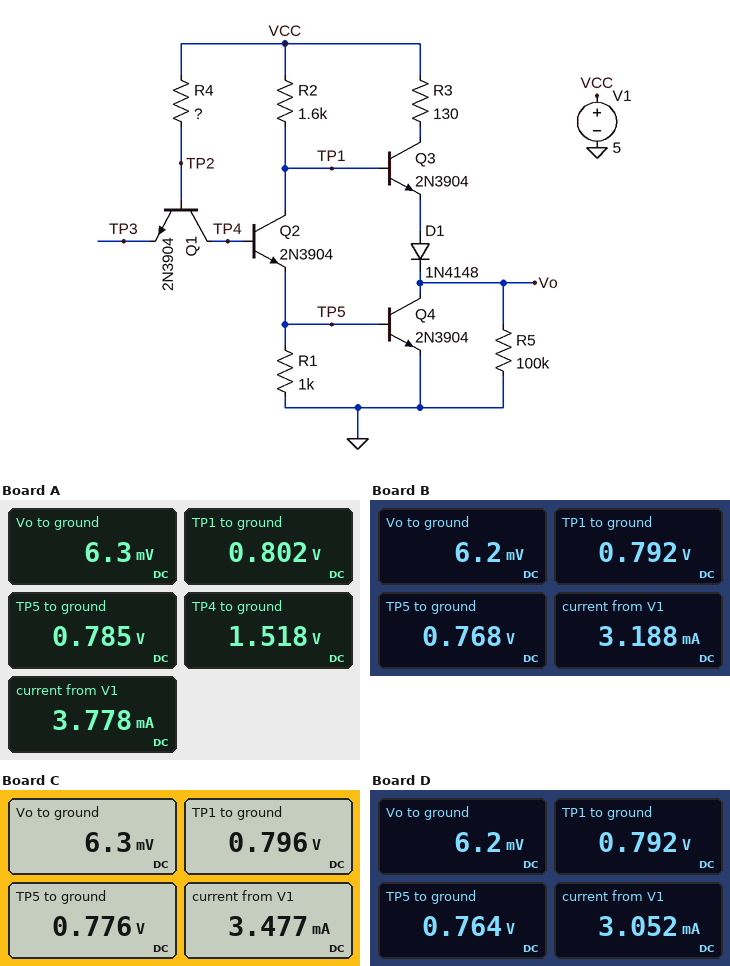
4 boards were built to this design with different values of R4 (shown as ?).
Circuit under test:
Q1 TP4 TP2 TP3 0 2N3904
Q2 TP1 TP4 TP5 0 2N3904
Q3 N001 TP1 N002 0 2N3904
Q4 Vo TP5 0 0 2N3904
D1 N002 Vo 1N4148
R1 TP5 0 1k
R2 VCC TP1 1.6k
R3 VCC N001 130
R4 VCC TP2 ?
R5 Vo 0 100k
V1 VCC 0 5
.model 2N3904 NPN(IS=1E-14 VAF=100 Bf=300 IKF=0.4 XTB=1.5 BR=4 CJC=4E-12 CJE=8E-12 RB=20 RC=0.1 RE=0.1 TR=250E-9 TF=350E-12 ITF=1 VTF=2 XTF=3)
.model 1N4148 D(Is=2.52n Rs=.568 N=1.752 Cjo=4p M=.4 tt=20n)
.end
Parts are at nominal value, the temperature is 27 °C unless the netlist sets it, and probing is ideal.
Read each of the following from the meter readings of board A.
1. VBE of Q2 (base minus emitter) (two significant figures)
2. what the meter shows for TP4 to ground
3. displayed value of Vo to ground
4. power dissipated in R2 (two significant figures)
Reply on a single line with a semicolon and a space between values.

730 mV; 1.518 V; 6.3 mV; 11 mW
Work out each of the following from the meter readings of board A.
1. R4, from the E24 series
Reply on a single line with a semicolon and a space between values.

2.4 kΩ
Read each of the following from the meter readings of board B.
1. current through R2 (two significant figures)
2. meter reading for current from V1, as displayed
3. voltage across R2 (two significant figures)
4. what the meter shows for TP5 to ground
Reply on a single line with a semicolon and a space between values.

2.6 mA; 3.188 mA; 4.2 V; 0.768 V
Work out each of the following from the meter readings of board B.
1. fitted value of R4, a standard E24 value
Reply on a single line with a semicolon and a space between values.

5.1 kΩ
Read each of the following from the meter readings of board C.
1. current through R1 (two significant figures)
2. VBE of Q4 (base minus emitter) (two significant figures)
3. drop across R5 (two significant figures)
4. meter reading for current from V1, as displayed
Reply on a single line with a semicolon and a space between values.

780 µA; 780 mV; 6.3 mV; 3.477 mA
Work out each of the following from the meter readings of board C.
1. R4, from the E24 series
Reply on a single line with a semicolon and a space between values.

3.3 kΩ
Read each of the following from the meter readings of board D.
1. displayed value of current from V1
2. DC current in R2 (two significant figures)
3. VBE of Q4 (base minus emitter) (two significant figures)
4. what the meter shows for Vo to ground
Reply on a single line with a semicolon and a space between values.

3.052 mA; 2.6 mA; 760 mV; 6.2 mV
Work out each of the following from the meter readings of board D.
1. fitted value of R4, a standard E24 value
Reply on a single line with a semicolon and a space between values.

6.8 kΩ
